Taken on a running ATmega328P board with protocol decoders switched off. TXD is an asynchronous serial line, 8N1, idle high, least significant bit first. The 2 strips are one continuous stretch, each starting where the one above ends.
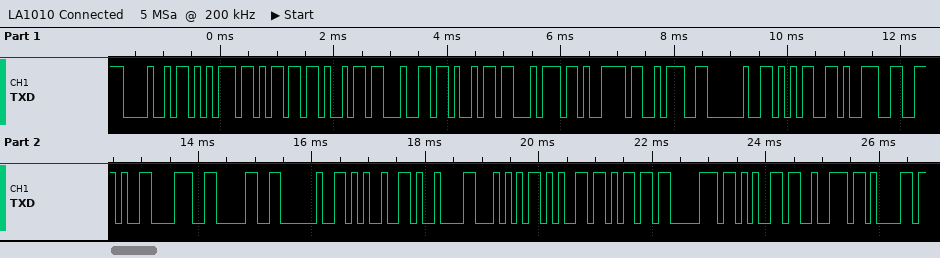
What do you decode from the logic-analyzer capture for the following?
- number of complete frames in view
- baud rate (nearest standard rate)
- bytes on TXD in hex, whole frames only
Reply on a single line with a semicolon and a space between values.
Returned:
25; 9600 baud; 48 75 6D 69 64 69 74 79 3A 20 35 39 2E 38 30 20 25 09 54 65 6D 70 65 72 61
